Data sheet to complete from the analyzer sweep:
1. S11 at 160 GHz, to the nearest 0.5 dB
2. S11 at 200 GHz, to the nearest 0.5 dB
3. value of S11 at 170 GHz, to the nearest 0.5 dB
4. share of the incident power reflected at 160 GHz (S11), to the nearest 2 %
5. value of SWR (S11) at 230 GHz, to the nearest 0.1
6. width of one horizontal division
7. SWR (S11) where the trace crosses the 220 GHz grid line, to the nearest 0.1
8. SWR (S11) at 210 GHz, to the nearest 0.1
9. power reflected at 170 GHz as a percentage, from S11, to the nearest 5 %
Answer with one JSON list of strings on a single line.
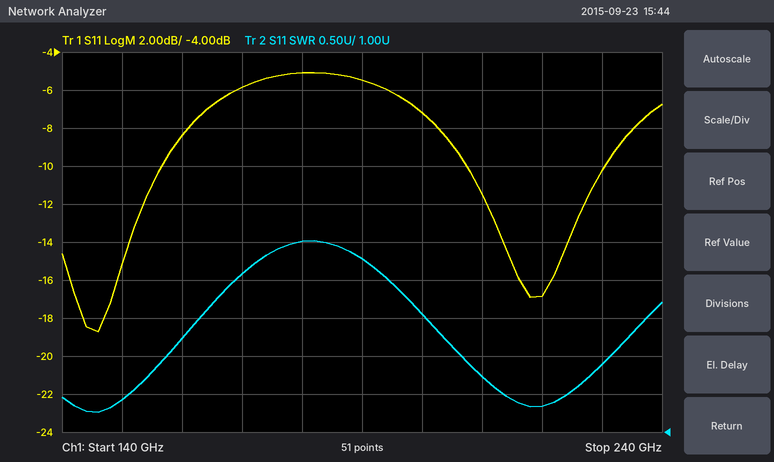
["-8.5 dB", "-7.0 dB", "-6.0 dB", "14 %", "1.9", "10 GHz", "1.3", "1.7", "25 %"]
